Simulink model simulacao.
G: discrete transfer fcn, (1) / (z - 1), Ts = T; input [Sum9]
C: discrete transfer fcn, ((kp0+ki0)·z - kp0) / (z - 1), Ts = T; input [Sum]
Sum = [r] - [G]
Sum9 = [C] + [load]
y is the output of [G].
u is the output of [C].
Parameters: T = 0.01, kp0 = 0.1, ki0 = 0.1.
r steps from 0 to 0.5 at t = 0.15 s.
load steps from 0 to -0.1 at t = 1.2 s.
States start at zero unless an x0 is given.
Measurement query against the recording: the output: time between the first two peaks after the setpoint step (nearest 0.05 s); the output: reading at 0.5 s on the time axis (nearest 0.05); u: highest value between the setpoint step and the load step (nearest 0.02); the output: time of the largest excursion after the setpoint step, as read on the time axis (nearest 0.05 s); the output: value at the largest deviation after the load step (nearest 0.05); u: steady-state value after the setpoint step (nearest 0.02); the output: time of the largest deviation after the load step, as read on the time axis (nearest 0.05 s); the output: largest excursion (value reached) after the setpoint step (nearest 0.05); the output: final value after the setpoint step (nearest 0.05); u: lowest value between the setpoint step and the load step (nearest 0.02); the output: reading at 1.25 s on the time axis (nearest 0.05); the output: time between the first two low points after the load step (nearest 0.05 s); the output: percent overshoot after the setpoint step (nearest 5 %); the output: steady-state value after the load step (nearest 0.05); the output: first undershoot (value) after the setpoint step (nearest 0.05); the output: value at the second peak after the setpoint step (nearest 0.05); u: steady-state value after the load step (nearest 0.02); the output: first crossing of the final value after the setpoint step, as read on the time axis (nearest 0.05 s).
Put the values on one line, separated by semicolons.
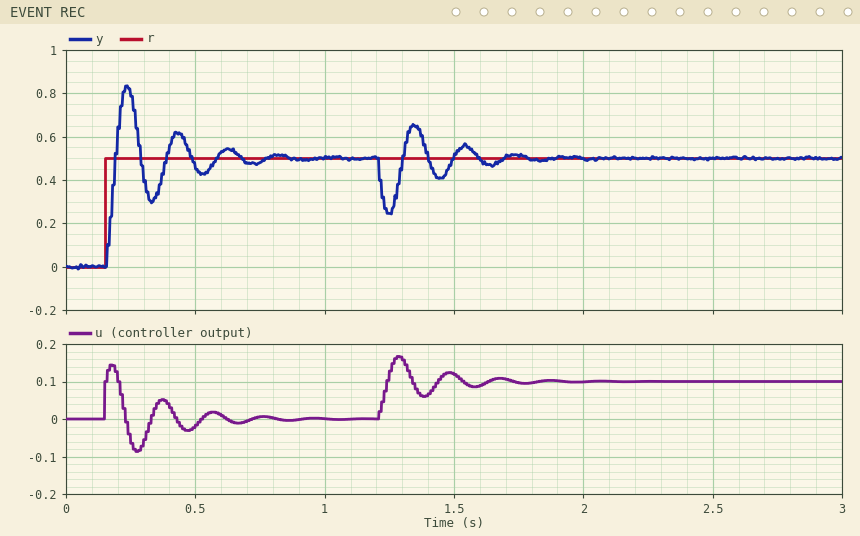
0.20 s; 0.45; 0.14; 0.25 s; 0.25; 0.00; 1.25 s; 0.85; 0.50; -0.08; 0.25; 0.20 s; 65 %; 0.50; 0.30; 0.60; 0.10; 0.20 s
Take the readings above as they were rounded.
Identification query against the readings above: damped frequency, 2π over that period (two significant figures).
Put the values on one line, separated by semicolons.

31 rad/s
